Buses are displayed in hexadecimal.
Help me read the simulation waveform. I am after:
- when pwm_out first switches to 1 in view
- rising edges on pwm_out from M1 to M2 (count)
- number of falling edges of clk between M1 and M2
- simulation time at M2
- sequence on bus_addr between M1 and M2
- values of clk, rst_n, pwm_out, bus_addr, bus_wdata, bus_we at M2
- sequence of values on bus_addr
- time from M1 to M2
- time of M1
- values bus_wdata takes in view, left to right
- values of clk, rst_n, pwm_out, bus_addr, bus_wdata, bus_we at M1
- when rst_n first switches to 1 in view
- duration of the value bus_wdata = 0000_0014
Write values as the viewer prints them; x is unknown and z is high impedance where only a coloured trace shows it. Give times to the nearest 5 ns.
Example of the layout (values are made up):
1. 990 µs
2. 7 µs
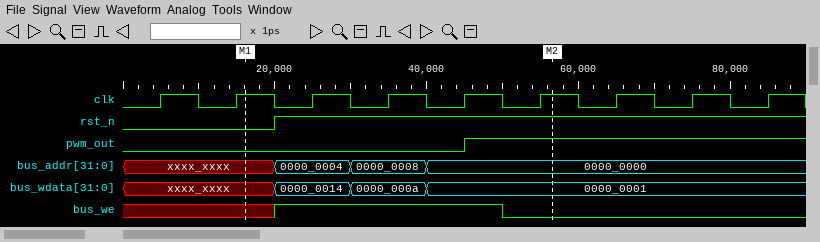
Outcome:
1. 45 ns
2. 1
3. 4
4. 55 ns
5. xxxx_xxxx, 0000_0004, 0000_0008, 0000_0000
6. clk=1, rst_n=1, pwm_out=1, bus_addr=0000_0000, bus_wdata=0000_0001, bus_we=0
7. xxxx_xxxx, 0000_0004, 0000_0008, 0000_0000
8. 40 ns
9. 15 ns
10. xxxx_xxxx, 0000_0014, 0000_000a, 0000_0001
11. clk=1, rst_n=0, pwm_out=0, bus_addr=xxxx_xxxx, bus_wdata=xxxx_xxxx, bus_we=x
12. 20 ns
13. 10 ns
